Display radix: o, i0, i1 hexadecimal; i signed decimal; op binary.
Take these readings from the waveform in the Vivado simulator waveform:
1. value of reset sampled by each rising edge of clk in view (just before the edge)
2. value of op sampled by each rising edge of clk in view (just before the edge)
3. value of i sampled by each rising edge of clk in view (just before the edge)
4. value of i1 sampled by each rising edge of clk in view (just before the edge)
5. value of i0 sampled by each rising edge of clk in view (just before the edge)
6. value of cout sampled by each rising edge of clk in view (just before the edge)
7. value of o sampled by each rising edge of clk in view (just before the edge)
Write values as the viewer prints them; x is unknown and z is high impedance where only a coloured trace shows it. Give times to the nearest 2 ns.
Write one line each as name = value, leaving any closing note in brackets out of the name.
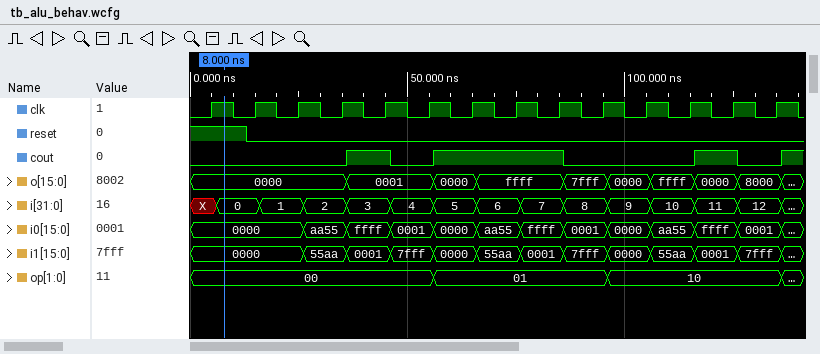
value of reset sampled by each rising edge of clk in view = 1 0 0 0 0 0 0 0 0 0 0 0 0 0
value of op sampled by each rising edge of clk in view = 00, 00, 00, 00, 00, 00, 01, 01, 01, 01, 10, 10, 10, 10
value of i sampled by each rising edge of clk in view = X, 0, 1, 2, 3, 4, 5, 6, 7, 8, 9, 10, 11, 12
value of i1 sampled by each rising edge of clk in view = 0000, 0000, 0000, 55aa, 0001, 7fff, 0000, 55aa, 0001, 7fff, 0000, 55aa, 0001, 7fff
value of i0 sampled by each rising edge of clk in view = 0000, 0000, 0000, aa55, ffff, 0001, 0000, aa55, ffff, 0001, 0000, aa55, ffff, 0001
value of cout sampled by each rising edge of clk in view = 0 0 0 0 1 0 1 1 1 0 0 0 1 0
value of o sampled by each rising edge of clk in view = 0000, 0000, 0000, 0000, 0001, 0001, 0000, ffff, ffff, 7fff, 0000, ffff, 0000, 8000
